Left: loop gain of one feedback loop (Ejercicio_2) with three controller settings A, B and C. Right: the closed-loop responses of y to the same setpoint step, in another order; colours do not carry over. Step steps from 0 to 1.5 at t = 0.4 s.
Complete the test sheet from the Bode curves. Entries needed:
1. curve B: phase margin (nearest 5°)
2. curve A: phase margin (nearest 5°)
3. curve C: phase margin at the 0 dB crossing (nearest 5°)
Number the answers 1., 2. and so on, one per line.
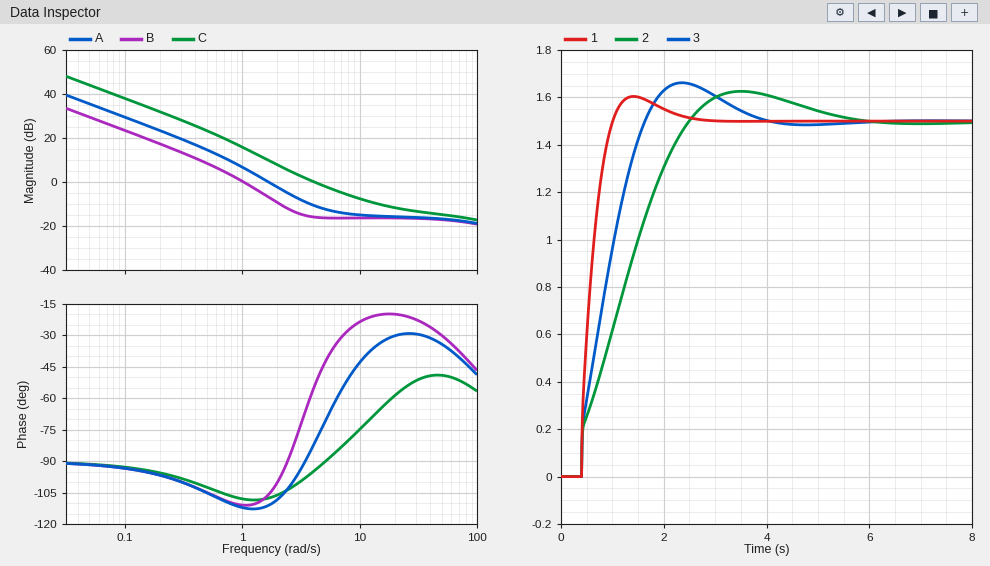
1. 70°
2. 70°
3. 85°
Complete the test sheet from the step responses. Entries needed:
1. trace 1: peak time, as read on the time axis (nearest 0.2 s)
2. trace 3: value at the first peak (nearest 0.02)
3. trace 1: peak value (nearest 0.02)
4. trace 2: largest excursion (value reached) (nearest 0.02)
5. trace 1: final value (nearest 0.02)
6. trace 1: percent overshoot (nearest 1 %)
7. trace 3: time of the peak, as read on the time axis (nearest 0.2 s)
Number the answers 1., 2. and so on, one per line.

1. 1.4 s
2. 1.66
3. 1.60
4. 1.62
5. 1.50
6. 7 %
7. 2.4 s
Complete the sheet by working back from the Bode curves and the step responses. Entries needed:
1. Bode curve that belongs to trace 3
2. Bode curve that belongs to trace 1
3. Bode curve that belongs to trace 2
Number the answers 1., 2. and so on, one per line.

1. A
2. C
3. B
